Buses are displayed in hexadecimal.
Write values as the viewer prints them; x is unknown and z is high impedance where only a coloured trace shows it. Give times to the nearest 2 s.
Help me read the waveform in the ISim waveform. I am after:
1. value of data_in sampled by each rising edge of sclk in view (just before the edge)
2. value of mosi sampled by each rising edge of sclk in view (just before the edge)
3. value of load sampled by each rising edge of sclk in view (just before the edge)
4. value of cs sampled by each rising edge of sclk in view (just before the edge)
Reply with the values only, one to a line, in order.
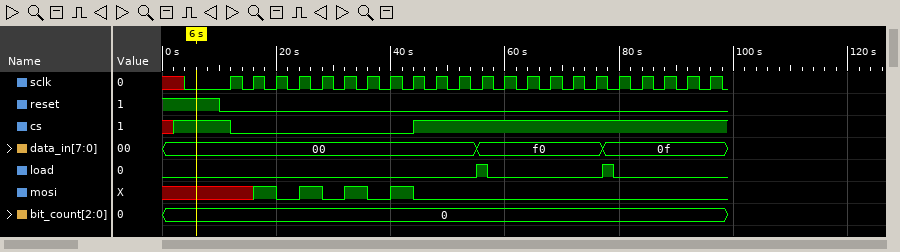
00, 00, 00, 00, 00, 00, 00, 00, 00, 00, 00, f0, f0, f0, f0, f0, f0, 0f, 0f, 0f, 0f, 0f
x x 1 0 1 0 1 0 1 0 0 0 0 0 0 0 0 0 0 0 0 0
0 0 0 0 0 0 0 0 0 0 0 1 0 0 0 0 0 0 0 0 0 0
1 0 0 0 0 0 0 0 0 1 1 1 1 1 1 1 1 1 1 1 1 1
